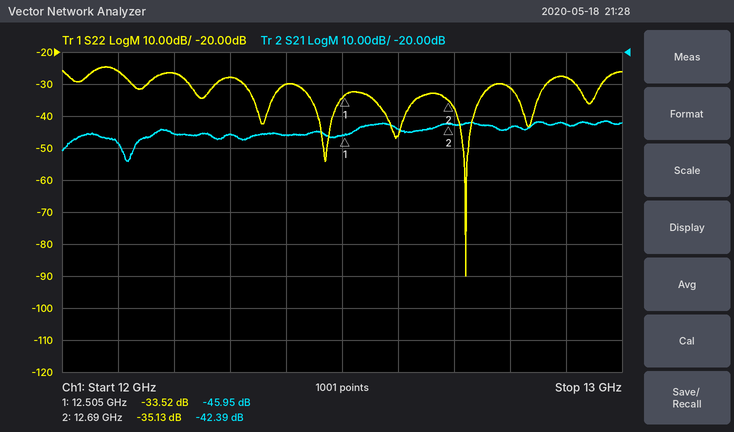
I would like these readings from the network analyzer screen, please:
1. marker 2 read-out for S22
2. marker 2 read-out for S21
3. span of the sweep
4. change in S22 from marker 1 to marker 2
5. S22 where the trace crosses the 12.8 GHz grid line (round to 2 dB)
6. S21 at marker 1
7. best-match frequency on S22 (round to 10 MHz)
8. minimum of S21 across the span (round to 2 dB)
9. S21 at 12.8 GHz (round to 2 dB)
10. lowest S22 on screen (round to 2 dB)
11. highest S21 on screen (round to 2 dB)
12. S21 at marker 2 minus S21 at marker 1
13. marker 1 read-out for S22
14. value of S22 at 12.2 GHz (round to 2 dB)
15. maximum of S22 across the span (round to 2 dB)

-35.13 dB
-42.39 dB
1 GHz
-1.61 dB
-32 dB
-45.95 dB
12.72 GHz
-54 dB
-44 dB
-90 dB
-42 dB
3.56 dB
-33.52 dB
-26 dB
-24 dB
